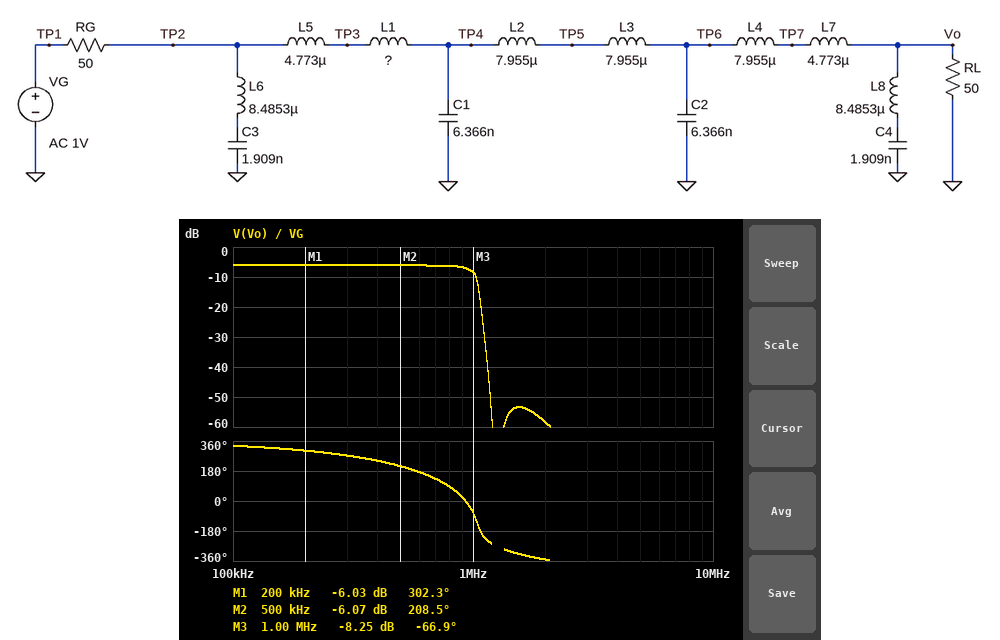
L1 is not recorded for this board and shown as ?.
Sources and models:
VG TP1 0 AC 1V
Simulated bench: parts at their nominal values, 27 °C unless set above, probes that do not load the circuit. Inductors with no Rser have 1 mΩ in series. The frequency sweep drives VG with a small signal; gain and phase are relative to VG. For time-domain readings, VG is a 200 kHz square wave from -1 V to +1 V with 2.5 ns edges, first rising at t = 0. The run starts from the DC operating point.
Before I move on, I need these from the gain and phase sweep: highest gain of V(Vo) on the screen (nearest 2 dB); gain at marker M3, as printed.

-6 dB
-8.25 dB
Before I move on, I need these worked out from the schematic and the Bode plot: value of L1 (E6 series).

4.7 µH
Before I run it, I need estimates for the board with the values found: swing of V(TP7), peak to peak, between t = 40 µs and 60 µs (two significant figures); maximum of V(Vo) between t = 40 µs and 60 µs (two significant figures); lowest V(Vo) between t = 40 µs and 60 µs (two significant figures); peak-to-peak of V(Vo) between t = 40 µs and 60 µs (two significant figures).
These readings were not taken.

1.3 V
730 mV
-730 mV
1.5 V
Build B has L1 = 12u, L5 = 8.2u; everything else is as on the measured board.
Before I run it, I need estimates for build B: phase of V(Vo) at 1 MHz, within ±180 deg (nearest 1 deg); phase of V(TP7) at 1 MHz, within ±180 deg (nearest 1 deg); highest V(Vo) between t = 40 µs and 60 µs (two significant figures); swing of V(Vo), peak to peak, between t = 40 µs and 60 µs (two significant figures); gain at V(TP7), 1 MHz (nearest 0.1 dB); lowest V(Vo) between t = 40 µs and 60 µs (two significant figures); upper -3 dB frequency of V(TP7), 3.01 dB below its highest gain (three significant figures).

-160 deg
-70 deg
660 mV
1.3 V
-23.9 dB
-660 mV
769 kHz
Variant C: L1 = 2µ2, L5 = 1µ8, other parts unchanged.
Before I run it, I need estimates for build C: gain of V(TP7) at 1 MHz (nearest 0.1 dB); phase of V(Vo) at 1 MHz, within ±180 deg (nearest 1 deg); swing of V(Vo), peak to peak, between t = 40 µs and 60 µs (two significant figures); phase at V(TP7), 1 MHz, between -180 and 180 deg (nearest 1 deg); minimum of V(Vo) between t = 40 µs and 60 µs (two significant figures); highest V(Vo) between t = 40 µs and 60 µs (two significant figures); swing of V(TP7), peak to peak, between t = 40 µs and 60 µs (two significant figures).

-20.5 dB
-18 deg
1.3 V
72 deg
-650 mV
650 mV
1.2 V
